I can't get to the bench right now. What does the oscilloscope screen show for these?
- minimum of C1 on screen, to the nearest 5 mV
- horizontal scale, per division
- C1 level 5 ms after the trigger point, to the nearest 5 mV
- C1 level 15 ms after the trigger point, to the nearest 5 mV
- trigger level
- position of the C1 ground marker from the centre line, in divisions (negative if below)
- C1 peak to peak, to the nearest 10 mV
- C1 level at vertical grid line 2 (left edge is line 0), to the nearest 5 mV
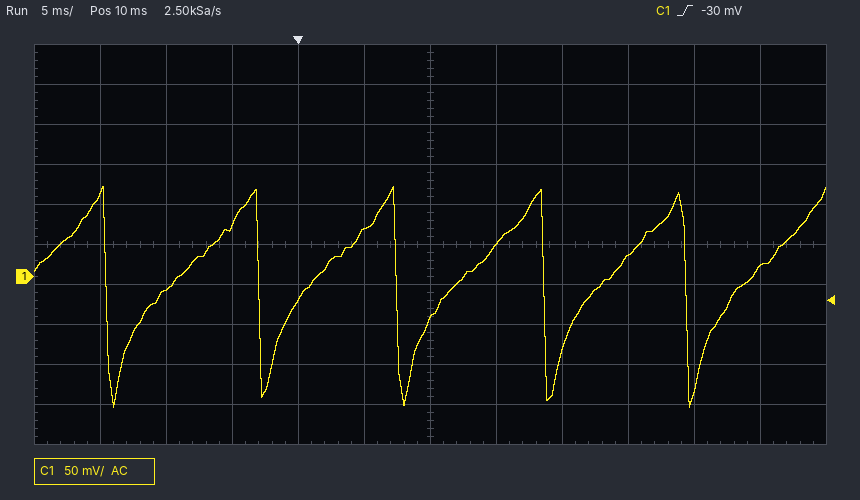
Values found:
-165 mV
5 ms
60 mV
40 mV
-30 mV
-0.8 div
280 mV
-15 mV
